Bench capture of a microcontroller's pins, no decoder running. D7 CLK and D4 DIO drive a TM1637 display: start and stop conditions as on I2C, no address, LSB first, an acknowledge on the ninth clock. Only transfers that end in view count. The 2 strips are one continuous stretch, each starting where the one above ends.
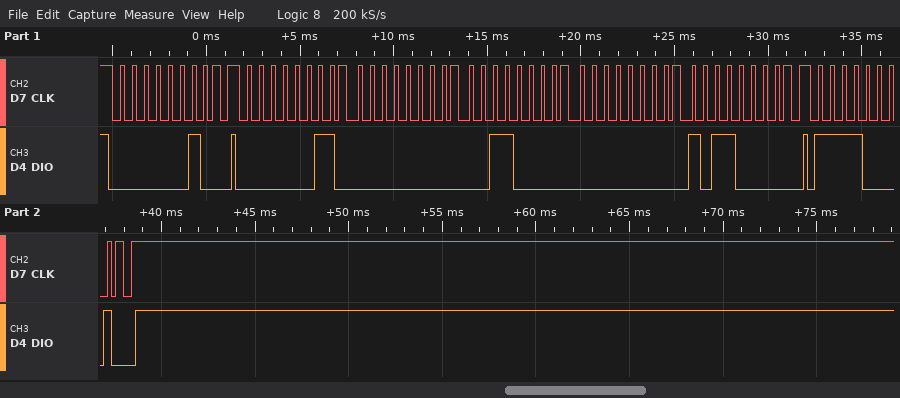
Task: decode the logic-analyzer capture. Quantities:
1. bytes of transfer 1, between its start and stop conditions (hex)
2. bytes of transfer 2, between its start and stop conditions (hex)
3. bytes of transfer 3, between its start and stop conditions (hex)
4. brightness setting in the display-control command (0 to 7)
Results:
40
C0 00 0C 00 0D
8F
7
